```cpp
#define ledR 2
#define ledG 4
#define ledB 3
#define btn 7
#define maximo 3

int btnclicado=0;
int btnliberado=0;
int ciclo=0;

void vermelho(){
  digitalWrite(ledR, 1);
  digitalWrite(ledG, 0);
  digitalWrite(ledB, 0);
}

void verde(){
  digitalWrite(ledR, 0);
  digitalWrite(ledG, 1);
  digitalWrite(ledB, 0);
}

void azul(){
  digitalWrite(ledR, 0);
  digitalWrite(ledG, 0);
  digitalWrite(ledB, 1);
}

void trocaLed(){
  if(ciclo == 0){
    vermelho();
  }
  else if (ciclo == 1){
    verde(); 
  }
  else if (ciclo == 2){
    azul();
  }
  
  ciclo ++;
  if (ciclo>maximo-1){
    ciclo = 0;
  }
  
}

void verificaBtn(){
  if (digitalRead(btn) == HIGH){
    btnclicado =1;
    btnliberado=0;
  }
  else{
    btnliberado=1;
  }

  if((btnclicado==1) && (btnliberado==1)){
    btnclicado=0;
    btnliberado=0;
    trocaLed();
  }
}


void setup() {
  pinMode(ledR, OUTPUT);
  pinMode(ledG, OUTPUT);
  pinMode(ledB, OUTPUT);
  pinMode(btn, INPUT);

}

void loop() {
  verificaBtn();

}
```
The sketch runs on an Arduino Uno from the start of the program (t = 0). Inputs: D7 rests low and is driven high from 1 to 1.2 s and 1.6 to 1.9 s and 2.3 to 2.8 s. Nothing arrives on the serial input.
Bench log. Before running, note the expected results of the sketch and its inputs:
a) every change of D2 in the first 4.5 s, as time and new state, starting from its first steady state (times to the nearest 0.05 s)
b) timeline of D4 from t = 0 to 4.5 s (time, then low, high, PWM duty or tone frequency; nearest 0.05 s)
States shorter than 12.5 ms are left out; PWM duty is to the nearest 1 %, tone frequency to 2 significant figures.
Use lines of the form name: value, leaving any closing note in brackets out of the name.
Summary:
every change of D2 in the first 4.5 s, as time and new state, starting from its first steady state: 0 s low; 1.2 s high; 1.9 s low
timeline of D4 from t = 0 to 4.5 s: 0 s low; 1.9 s high; 2.8 s low
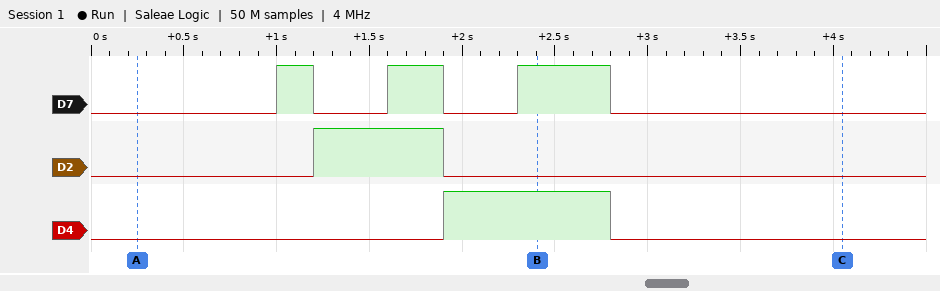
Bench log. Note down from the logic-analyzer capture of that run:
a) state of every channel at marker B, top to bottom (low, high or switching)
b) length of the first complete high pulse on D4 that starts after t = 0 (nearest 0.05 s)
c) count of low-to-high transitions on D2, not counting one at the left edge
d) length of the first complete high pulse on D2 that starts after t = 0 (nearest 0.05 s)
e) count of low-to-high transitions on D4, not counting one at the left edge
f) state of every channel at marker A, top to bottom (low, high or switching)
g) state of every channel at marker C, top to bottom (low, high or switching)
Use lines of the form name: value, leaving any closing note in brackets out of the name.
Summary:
state of every channel at marker B, top to bottom: D7 high, D2 low, D4 high
length of the first complete high pulse on D4 that starts after t = 0: 0.90 s
count of low-to-high transitions on D2, not counting one at the left edge: 1
length of the first complete high pulse on D2 that starts after t = 0: 0.70 s
count of low-to-high transitions on D4, not counting one at the left edge: 1
state of every channel at marker A, top to bottom: D7 low, D2 low, D4 low
state of every channel at marker C, top to bottom: D7 low, D2 low, D4 low
